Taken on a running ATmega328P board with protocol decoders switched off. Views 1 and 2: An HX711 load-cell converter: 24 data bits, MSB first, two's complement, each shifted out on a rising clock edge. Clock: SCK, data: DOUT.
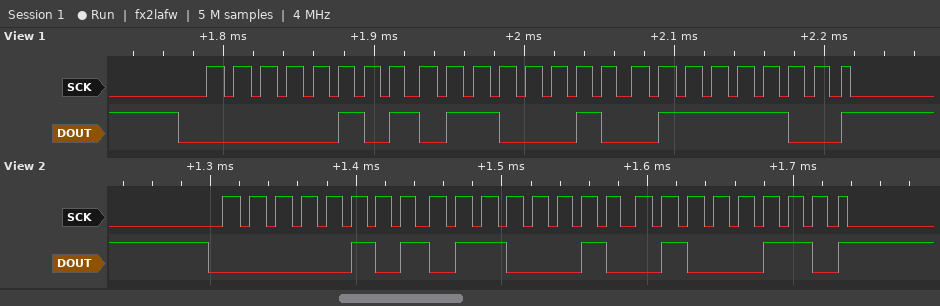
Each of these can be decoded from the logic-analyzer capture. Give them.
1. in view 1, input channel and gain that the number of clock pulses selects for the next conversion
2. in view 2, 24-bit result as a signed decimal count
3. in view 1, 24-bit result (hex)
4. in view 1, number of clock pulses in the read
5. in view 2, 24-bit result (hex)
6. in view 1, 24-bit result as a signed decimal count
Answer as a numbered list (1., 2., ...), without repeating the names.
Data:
1. channel A, gain 128
2. 352838
3. 0x05627C
4. 25
5. 0x056246
6. 352892
